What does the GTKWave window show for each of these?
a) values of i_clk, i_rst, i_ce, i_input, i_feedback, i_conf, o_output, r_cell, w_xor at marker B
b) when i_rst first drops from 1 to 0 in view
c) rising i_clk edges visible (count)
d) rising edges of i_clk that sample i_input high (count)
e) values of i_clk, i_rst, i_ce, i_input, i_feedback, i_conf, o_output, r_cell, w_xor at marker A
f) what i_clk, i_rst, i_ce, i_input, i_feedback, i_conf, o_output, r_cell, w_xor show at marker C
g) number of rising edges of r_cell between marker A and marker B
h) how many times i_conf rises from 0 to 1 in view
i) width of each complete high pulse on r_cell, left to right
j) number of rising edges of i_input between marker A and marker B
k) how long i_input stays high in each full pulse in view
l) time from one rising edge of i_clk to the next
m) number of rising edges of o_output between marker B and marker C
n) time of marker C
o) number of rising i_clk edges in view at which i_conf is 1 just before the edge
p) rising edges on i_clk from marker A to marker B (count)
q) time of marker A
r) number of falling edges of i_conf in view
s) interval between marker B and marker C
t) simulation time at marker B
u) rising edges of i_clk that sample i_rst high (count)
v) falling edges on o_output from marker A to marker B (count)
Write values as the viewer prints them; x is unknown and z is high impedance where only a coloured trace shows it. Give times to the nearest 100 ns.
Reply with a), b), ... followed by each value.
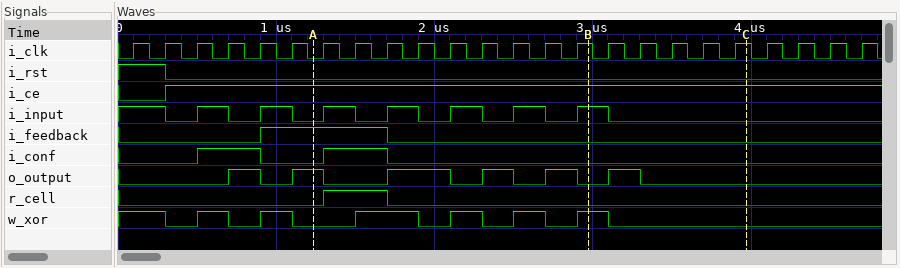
a) i_clk=1, i_rst=0, i_ce=1, i_input=1, i_feedback=0, i_conf=0, o_output=0, r_cell=0, w_xor=1
b) 300 ns
c) 24
d) 9
e) i_clk=0, i_rst=0, i_ce=1, i_input=0, i_feedback=1, i_conf=0, o_output=1, r_cell=0, w_xor=0
f) i_clk=1, i_rst=0, i_ce=1, i_input=0, i_feedback=0, i_conf=0, o_output=0, r_cell=0, w_xor=0
g) 1
h) 2
i) 400 ns
j) 5
k) 200 ns, 200 ns, 200 ns, 200 ns, 200 ns, 200 ns, 200 ns
l) 200 ns
m) 1
n) 4000 ns
o) 4
p) 9
q) 1200 ns
r) 2
s) 1000 ns
t) 3000 ns
u) 2
v) 4
